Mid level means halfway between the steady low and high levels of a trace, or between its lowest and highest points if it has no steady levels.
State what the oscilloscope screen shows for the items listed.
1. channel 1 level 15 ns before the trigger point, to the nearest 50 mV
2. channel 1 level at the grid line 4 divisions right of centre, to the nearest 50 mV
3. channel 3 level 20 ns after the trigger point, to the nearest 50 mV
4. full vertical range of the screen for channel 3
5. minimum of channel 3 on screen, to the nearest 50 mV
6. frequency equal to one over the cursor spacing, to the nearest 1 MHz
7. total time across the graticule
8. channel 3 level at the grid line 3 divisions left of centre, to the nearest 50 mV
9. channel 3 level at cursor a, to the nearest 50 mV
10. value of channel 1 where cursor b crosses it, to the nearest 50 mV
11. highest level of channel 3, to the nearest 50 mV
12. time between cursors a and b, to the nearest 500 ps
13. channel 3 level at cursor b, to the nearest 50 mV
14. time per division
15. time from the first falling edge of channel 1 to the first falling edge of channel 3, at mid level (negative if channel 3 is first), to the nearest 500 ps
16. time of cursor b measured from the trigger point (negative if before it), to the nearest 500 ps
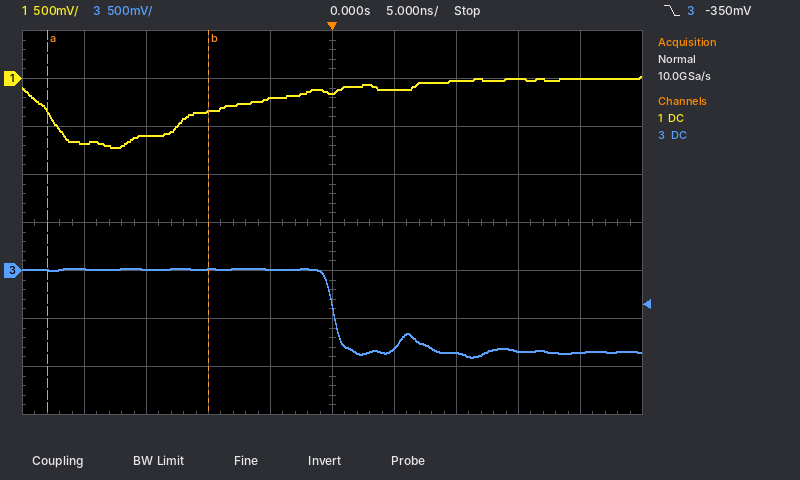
-600 mV
0 mV
-850 mV
4 V
-900 mV
77 MHz
50 ns
0 mV
0 mV
-350 mV
0 mV
13.0 ns
0 mV
5 ns
+23.0 ns
-10.0 ns
